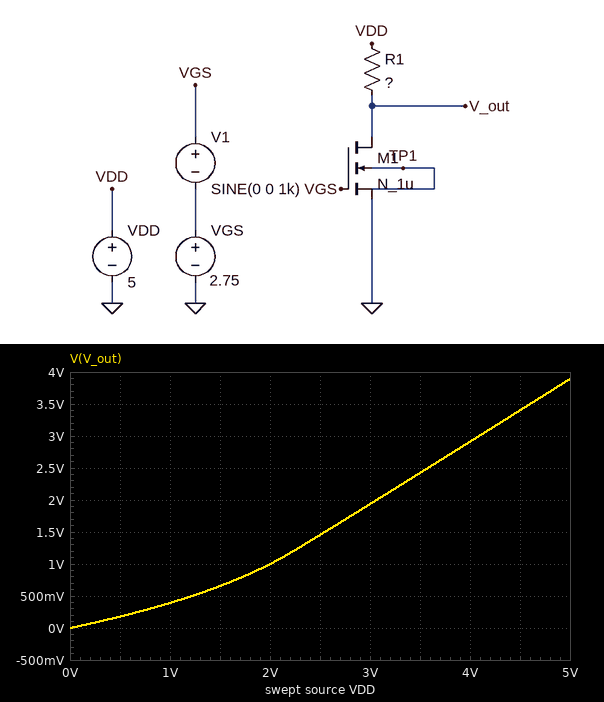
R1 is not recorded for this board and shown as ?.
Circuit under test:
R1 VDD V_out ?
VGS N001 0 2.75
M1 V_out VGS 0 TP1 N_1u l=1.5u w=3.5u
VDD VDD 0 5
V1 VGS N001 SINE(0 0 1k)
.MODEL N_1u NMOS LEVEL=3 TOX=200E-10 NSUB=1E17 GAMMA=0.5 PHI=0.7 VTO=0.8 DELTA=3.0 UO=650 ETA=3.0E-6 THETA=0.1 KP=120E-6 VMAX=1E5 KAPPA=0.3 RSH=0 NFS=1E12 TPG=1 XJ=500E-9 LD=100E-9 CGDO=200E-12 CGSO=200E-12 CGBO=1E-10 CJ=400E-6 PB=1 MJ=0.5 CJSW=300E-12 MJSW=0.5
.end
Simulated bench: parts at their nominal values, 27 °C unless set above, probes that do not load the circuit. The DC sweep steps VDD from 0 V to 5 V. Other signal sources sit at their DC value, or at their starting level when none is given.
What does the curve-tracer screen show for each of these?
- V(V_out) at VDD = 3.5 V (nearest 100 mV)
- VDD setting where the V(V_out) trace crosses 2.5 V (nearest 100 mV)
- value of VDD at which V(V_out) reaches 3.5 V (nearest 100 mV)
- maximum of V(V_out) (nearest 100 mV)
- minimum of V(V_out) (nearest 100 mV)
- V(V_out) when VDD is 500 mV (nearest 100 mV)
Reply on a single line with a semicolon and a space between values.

2.4 V; 3.6 V; 4.6 V; 3.9 V; 0 V; 200 mV
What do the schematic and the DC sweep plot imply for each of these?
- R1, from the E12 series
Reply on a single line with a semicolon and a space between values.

3.9 kΩ
